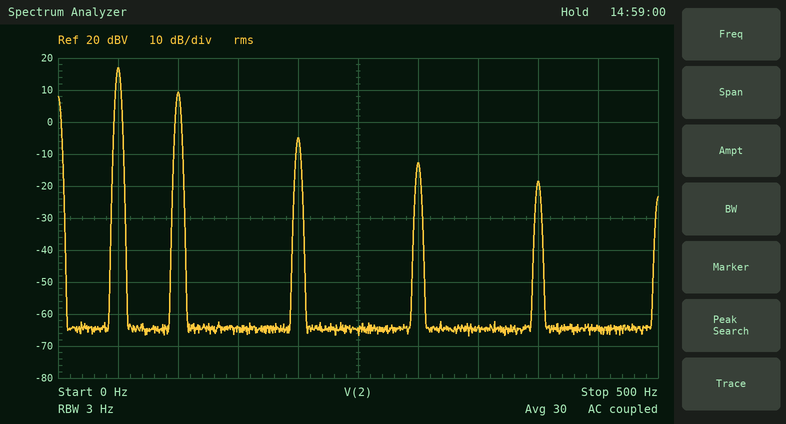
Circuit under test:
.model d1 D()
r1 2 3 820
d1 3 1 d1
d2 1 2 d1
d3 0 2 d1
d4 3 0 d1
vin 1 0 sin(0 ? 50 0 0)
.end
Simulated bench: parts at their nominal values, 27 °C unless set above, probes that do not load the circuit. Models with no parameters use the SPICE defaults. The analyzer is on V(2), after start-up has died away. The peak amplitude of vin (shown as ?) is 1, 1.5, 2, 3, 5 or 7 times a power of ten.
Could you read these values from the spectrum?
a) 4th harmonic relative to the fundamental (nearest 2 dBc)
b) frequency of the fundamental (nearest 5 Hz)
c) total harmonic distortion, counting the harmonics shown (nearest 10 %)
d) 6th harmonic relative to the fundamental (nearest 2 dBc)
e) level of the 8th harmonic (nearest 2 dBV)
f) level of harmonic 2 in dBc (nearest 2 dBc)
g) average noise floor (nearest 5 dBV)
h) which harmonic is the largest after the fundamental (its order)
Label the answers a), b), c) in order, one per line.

a) -22 dBc
b) 50 Hz
c) 40 %
d) -30 dBc
e) -18 dBV
f) -8 dBc
g) -65 dBV
h) 2
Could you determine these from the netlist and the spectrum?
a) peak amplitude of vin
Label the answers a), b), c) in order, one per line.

a) 20 V
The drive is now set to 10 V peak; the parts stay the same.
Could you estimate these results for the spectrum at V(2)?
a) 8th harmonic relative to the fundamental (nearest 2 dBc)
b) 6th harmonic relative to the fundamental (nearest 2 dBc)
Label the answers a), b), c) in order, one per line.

a) -40 dBc
b) -32 dBc
